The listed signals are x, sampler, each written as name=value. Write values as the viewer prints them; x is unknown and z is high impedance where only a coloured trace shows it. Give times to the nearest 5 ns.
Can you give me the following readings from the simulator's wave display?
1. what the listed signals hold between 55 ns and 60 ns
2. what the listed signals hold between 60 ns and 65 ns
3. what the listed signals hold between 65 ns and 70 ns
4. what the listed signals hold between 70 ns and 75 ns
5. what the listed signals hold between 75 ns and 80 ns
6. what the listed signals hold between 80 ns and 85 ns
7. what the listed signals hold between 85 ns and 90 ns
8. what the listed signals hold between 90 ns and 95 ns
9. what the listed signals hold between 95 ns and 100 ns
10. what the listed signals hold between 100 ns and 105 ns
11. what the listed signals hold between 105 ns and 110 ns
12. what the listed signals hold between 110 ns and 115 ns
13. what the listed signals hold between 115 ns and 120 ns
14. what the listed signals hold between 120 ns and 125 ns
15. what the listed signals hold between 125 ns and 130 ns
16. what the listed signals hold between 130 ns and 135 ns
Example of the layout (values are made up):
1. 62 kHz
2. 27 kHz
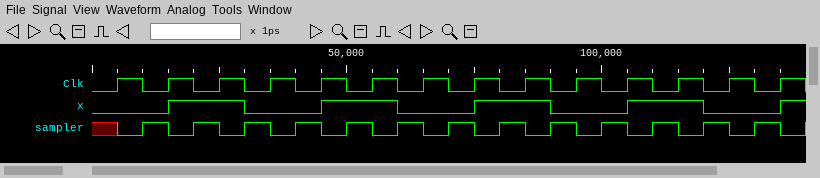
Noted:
1. x=1, sampler=0
2. x=0, sampler=1
3. x=0, sampler=0
4. x=0, sampler=1
5. x=1, sampler=0
6. x=1, sampler=1
7. x=1, sampler=0
8. x=0, sampler=1
9. x=0, sampler=0
10. x=0, sampler=1
11. x=1, sampler=0
12. x=1, sampler=1
13. x=1, sampler=0
14. x=0, sampler=1
15. x=0, sampler=0
16. x=0, sampler=1
